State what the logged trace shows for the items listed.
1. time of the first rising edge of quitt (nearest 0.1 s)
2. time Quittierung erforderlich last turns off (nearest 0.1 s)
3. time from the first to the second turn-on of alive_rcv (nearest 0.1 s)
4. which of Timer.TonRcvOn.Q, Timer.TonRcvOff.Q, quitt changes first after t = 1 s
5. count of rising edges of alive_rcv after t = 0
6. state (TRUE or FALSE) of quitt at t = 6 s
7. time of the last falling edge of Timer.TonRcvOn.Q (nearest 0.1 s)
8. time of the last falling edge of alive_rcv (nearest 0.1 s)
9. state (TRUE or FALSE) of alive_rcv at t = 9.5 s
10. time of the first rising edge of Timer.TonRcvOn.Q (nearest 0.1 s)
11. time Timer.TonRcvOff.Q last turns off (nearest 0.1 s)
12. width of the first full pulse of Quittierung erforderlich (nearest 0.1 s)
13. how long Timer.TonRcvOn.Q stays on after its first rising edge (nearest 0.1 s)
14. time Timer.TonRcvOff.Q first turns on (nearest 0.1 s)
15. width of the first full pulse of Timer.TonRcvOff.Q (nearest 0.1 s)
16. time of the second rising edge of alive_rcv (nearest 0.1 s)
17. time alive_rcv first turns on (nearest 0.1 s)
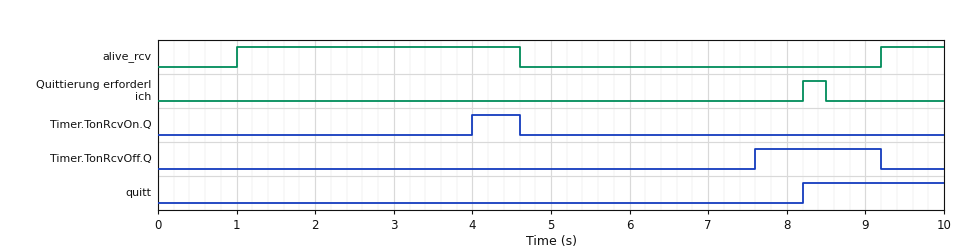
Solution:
8.2 s
8.5 s
8.2 s
Timer.TonRcvOn.Q
2
FALSE
4.6 s
4.6 s
TRUE
4.0 s
9.2 s
0.3 s
0.6 s
7.6 s
1.6 s
9.2 s
1.0 s
